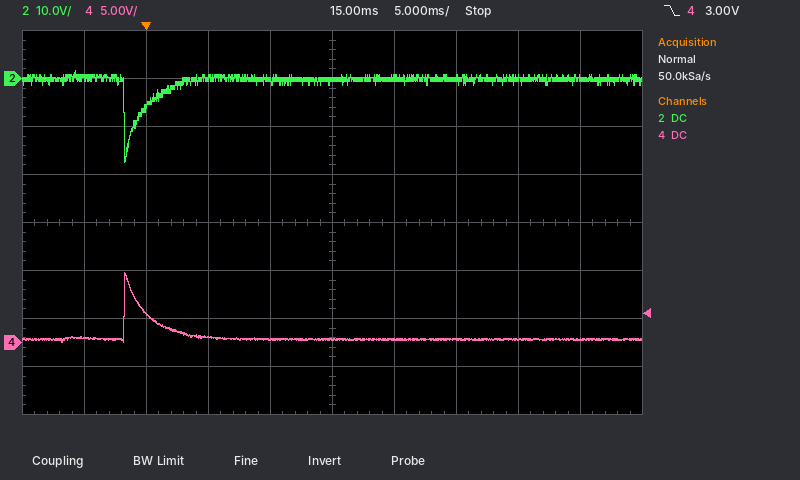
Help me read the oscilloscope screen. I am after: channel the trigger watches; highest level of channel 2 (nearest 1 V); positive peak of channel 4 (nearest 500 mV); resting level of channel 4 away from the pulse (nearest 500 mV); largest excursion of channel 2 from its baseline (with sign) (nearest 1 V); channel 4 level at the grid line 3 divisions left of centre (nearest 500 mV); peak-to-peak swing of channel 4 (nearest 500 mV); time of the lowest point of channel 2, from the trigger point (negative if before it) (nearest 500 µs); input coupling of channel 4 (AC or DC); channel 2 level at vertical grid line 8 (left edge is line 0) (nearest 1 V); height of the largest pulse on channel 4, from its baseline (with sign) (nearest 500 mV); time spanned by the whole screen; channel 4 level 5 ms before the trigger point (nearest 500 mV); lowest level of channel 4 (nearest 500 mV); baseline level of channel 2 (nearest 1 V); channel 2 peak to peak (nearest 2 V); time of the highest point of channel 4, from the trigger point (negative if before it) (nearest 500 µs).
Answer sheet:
channel 4
2 V
7.5 V
500 mV
-17 V
3.0 V
7.5 V
-1.5 ms
DC
0 V
+7.0 V
50 ms
500 mV
0.0 V
0 V
20 V
-1.5 ms
